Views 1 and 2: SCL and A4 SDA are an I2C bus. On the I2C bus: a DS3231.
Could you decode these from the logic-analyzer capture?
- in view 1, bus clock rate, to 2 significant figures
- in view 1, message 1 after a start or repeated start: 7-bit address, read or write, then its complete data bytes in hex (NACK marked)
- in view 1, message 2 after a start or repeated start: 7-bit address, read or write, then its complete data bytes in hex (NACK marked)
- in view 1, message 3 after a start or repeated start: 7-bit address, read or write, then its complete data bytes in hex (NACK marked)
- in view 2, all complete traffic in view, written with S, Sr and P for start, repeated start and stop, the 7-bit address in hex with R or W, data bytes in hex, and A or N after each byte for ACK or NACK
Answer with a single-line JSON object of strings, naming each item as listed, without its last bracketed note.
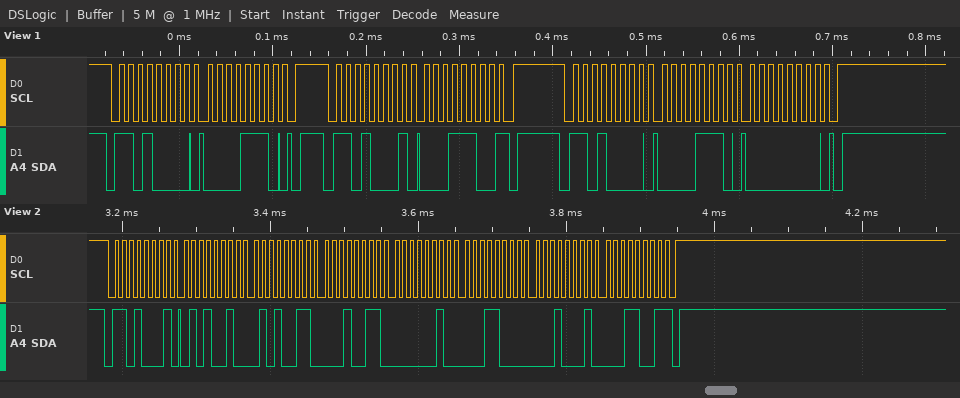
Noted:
{"in view 1, bus clock rate, to 2 significant figures": "100 kHz", "in view 1, message 1 after a start or repeated start: 7-bit address, read or write, then its complete data bytes in hex": "0x68 write: 0E", "in view 1, message 2 after a start or repeated start: 7-bit address, read or write, then its complete data bytes in hex": "0x68 read: 1C NACK", "in view 1, message 3 after a start or repeated start: 7-bit address, read or write, then its complete data bytes in hex": "0x68 write: 0E 00", "in view 2, all complete traffic in view, written with S, Sr and P for start, repeated start and stop, the 7-bit address in hex with R or W, data bytes in hex, and A or N after each byte for ACK or NACK": "S 68R A 52 A 53 A 13 A 02 A 18 A 11 A 19 N P"}
